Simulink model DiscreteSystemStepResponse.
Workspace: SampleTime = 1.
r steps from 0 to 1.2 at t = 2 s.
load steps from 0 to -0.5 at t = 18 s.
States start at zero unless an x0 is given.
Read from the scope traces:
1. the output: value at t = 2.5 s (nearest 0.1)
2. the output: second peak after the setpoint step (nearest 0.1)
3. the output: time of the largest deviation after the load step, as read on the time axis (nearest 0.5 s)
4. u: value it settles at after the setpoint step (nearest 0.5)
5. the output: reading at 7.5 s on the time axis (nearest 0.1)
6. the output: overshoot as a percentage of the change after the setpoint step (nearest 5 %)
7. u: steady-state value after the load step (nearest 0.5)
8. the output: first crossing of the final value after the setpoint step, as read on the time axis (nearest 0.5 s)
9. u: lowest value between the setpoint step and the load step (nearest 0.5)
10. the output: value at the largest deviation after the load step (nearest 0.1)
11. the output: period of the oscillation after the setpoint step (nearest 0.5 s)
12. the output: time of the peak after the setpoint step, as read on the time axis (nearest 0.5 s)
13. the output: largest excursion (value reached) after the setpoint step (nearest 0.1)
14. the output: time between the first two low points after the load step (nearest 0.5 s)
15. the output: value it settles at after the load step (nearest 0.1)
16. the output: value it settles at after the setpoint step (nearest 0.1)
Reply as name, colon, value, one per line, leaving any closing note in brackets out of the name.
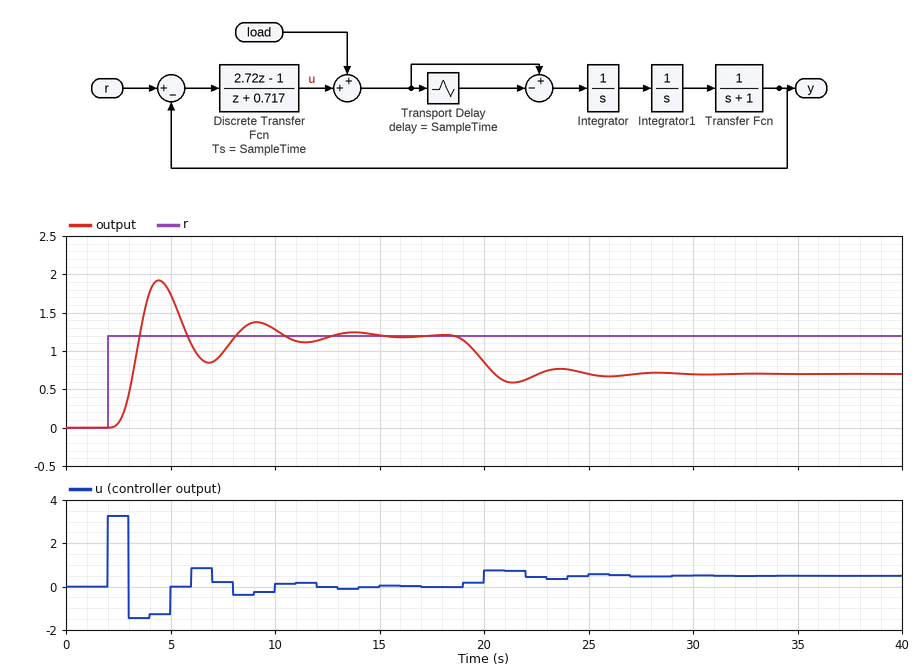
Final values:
the output: value at t = 2.5 s: 0.1
the output: second peak after the setpoint step: 1.4
the output: time of the largest deviation after the load step, as read on the time axis: 21.5 s
u: value it settles at after the setpoint step: 0.0
the output: reading at 7.5 s on the time axis: 1.0
the output: overshoot as a percentage of the change after the setpoint step: 60 %
u: steady-state value after the load step: 0.5
the output: first crossing of the final value after the setpoint step, as read on the time axis: 3.5 s
u: lowest value between the setpoint step and the load step: -1.5
the output: value at the largest deviation after the load step: 0.6
the output: period of the oscillation after the setpoint step: 4.5 s
the output: time of the peak after the setpoint step, as read on the time axis: 4.5 s
the output: largest excursion (value reached) after the setpoint step: 1.9
the output: time between the first two low points after the load step: 4.5 s
the output: value it settles at after the load step: 0.7
the output: value it settles at after the setpoint step: 1.2
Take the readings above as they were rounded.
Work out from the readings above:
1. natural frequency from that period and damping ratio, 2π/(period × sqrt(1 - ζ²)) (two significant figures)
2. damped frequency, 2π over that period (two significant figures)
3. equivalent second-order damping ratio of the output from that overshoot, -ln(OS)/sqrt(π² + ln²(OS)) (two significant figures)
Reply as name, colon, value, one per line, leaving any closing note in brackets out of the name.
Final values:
natural frequency from that period and damping ratio, 2π/(period × sqrt(1 - ζ²)): 1.4 rad/s
damped frequency, 2π over that period: 1.4 rad/s
equivalent second-order damping ratio of the output from that overshoot, -ln(OS)/sqrt(π² + ln²(OS)): 0.16
